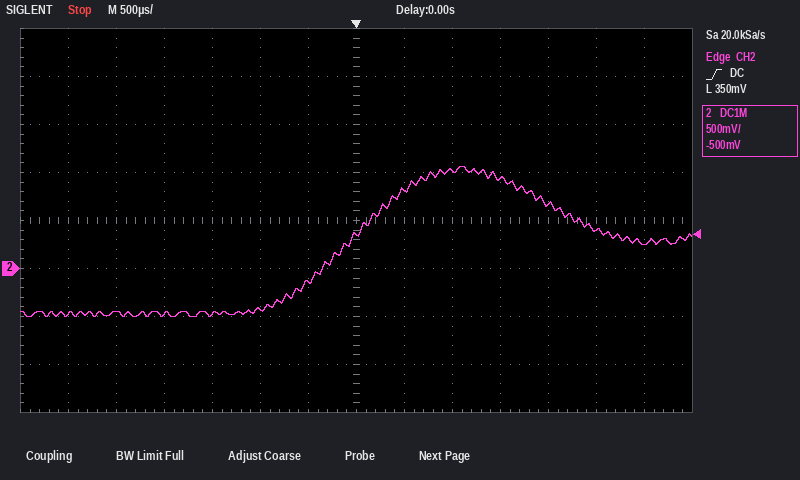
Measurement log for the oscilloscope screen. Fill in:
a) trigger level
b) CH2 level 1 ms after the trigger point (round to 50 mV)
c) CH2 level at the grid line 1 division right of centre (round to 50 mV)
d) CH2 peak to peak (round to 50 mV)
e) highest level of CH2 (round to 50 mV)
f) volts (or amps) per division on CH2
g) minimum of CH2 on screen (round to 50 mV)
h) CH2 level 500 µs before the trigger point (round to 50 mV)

350 mV
1.00 V
800 mV
1.55 V
1.05 V
500 mV
-500 mV
-150 mV
